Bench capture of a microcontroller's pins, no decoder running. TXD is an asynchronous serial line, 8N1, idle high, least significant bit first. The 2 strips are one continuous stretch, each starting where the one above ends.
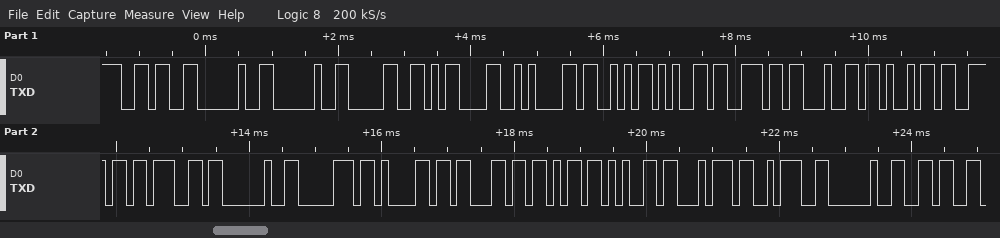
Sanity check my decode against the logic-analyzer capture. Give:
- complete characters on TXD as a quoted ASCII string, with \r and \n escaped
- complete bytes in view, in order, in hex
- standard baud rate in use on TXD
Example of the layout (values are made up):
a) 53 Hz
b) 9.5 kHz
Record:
a) "6  0\r\nSending packet: 6"
b) 36 20 20 30 0D 0A 53 65 6E 64 69 6E 67 20 70 61 63 6B 65 74 3A 20 36
c) 9600 baud
